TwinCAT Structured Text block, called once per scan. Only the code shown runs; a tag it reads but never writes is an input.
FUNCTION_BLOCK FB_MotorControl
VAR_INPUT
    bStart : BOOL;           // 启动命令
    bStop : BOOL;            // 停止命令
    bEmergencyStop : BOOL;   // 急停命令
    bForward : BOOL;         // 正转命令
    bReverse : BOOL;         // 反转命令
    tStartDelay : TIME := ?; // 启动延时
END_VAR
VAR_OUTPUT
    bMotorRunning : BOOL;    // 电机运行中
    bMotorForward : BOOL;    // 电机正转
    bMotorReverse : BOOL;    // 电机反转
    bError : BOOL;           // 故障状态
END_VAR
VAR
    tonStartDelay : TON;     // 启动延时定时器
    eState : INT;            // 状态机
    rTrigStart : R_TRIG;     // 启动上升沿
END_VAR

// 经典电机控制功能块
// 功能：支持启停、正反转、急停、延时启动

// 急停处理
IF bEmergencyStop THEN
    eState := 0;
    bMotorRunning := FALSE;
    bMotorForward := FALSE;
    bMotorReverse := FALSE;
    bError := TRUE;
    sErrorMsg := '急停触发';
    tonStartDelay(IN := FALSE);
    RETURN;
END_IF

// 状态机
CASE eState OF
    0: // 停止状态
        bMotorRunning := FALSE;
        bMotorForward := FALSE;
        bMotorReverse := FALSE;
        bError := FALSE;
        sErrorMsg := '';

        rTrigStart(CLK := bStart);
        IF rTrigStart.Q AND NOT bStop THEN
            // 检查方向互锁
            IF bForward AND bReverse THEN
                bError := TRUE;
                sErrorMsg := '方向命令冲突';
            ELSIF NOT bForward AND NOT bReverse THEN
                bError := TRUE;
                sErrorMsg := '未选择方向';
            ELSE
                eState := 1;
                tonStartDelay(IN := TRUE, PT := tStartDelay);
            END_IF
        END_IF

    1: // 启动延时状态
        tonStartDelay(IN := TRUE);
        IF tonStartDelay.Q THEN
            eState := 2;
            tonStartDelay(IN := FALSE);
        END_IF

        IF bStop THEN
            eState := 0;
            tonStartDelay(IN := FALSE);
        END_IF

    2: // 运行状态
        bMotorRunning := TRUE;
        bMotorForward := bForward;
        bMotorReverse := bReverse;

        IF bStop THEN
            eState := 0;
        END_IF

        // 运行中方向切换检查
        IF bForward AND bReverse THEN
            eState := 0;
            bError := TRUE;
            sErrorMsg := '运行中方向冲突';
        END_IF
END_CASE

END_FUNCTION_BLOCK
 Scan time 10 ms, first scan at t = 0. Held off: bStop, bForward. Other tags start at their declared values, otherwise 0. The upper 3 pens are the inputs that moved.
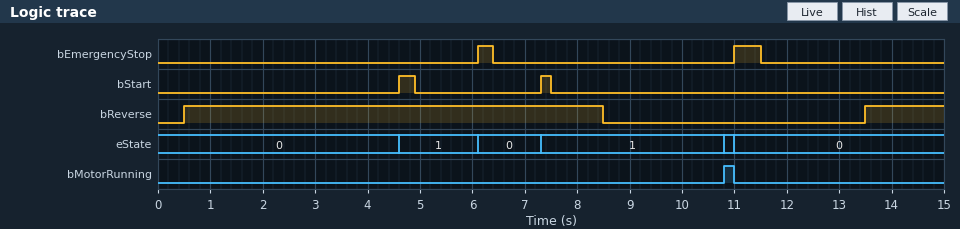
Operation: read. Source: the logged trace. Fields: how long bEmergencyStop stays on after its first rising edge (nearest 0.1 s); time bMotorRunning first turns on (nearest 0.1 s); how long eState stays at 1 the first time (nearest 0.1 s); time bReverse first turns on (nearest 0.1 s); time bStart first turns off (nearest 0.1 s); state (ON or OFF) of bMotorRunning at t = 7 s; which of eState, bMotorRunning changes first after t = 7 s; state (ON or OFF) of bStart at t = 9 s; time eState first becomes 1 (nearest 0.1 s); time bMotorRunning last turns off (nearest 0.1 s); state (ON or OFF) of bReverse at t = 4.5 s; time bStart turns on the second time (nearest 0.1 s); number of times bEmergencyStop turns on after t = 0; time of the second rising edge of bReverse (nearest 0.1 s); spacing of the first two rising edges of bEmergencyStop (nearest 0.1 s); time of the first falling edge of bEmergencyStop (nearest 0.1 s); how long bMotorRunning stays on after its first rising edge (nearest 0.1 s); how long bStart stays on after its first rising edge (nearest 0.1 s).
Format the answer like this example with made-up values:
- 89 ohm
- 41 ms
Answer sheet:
- 0.3 s
- 10.8 s
- 1.5 s
- 0.5 s
- 4.9 s
- OFF
- eState
- OFF
- 4.6 s
- 11.0 s
- ON
- 7.3 s
- 2
- 13.5 s
- 4.9 s
- 6.4 s
- 0.2 s
- 0.3 s
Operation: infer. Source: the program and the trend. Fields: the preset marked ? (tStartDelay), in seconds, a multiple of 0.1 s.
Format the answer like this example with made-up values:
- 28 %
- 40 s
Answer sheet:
- 3.5 s
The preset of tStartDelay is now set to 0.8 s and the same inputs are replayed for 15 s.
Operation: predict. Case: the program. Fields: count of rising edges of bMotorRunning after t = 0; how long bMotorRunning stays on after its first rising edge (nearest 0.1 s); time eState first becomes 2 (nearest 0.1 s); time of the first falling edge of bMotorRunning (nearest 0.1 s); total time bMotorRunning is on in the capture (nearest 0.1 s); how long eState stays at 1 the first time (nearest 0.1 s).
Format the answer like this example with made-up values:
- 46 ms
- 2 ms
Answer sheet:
- 2
- 0.7 s
- 5.4 s
- 6.1 s
- 3.6 s
- 0.8 s
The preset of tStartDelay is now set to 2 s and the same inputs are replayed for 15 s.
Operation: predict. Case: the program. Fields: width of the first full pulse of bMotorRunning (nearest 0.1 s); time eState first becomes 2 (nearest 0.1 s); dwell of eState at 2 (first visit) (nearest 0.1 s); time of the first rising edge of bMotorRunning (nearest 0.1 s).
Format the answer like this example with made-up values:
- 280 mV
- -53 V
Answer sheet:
- 1.7 s
- 9.3 s
- 1.7 s
- 9.3 s
